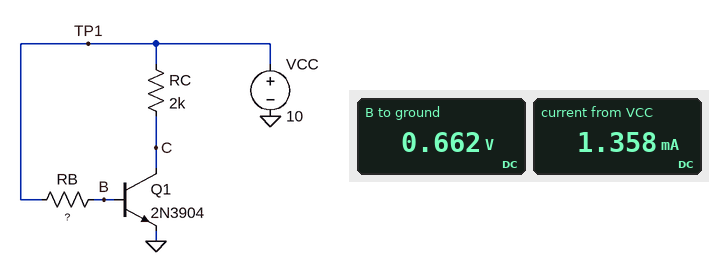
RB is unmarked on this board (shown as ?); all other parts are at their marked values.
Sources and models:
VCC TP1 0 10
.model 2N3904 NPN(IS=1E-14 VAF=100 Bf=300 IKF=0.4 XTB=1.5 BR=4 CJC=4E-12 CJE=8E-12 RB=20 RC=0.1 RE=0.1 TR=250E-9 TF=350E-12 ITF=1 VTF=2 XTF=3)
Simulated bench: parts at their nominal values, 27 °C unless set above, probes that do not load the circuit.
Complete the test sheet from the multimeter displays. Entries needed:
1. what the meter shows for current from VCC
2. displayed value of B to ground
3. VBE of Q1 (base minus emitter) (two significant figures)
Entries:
1.358 mA
0.662 V
660 mV
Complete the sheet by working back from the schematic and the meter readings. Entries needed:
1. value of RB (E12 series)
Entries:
2.2 MΩ
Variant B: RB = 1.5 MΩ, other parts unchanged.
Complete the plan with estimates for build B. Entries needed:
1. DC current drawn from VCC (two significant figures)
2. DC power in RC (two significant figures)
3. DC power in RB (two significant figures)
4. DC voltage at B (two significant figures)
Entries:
2.0 mA
7.7 mW
58 µW
670 mV
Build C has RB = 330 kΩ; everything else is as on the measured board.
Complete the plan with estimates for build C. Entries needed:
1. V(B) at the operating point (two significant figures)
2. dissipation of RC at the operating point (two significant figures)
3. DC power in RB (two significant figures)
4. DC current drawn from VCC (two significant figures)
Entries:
700 mV
49 mW
260 µW
5.0 mA
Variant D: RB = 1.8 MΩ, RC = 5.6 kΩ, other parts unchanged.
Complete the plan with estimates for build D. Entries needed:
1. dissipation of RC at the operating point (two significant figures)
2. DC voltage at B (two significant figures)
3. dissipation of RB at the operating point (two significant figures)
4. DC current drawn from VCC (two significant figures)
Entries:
14 mW
670 mV
48 µW
1.6 mA
